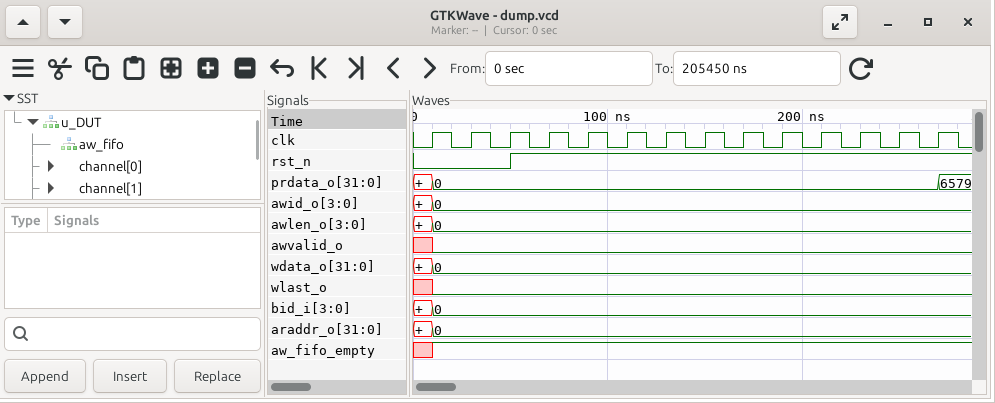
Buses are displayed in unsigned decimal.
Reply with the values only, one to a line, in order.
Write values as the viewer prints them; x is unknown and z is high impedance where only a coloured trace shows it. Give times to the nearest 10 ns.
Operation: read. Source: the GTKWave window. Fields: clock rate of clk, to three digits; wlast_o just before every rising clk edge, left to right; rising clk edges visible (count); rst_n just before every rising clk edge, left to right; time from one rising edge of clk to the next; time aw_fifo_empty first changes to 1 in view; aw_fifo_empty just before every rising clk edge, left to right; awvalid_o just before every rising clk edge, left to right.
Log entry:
50.0 MHz
x 0 0 0 0 0 0 0 0 0 0 0 0 0
14
0 0 0 1 1 1 1 1 1 1 1 1 1 1
20 ns
10 ns
x 1 1 1 1 1 1 1 1 1 1 1 1 1
x 0 0 0 0 0 0 0 0 0 0 0 0 0
